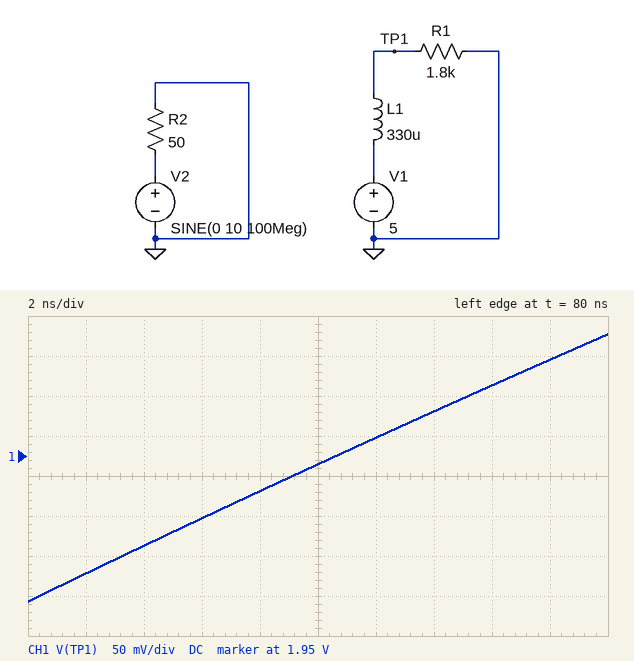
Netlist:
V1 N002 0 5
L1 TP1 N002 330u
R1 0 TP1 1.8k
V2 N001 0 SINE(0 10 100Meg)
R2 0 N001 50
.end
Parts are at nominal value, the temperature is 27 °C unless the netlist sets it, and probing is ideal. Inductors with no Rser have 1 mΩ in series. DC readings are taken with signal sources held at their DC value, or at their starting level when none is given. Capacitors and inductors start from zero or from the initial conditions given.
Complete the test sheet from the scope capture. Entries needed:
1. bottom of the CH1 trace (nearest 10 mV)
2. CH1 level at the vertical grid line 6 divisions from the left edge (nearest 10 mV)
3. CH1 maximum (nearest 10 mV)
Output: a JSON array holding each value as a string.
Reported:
["1.77 V", "1.97 V", "2.10 V"]
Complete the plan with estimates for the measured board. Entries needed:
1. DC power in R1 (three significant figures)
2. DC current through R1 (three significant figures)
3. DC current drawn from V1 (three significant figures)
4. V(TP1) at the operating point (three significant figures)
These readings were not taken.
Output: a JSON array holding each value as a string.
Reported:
["13.9 mW", "2.78 mA", "2.78 mA", "5.00 V"]
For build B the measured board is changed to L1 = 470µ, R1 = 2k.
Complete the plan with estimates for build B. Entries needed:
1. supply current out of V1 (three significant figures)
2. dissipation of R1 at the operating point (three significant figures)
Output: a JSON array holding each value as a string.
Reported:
["2.50 mA", "12.5 mW"]
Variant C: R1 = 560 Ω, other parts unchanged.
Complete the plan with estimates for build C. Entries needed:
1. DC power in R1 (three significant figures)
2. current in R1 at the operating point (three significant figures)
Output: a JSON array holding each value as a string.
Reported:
["44.6 mW", "8.93 mA"]
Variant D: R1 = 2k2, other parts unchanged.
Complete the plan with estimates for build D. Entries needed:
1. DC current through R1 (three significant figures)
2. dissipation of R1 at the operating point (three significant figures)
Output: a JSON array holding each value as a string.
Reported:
["2.27 mA", "11.4 mW"]
